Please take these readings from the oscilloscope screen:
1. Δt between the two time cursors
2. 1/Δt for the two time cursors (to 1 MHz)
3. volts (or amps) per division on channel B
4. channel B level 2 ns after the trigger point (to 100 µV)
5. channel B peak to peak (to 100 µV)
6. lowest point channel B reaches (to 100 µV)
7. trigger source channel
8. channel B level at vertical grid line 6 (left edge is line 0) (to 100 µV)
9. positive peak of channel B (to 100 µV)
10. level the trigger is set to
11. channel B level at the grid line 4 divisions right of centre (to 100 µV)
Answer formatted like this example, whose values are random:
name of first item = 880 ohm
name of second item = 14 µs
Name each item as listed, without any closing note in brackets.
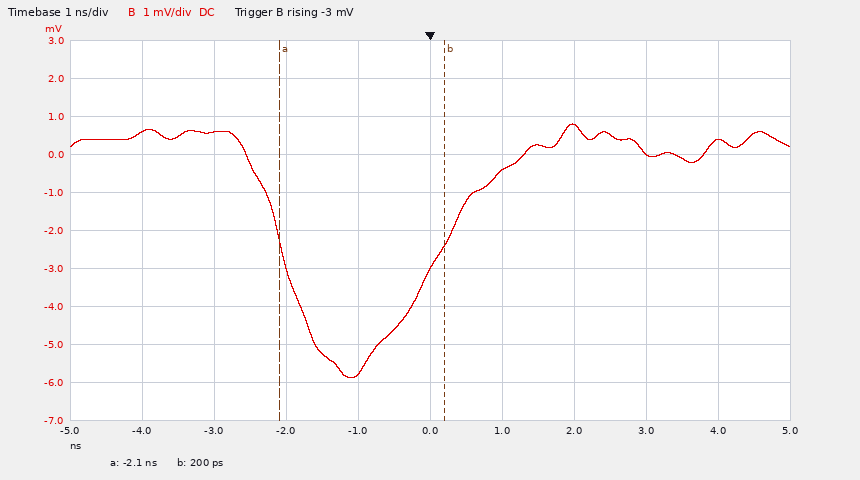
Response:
Δt between the two time cursors = 2.3 ns
1/Δt for the two time cursors = 435 MHz
volts (or amps) per division on channel B = 1 mV
channel B level 2 ns after the trigger point = 800 µV
channel B peak to peak = 6.7 mV
lowest point channel B reaches = -5.9 mV
trigger source channel = channel B
channel B level at vertical grid line 6 (left edge is line 0) = -400 µV
positive peak of channel B = 800 µV
level the trigger is set to = -3 mV
channel B level at the grid line 4 divisions right of centre = 400 µV
